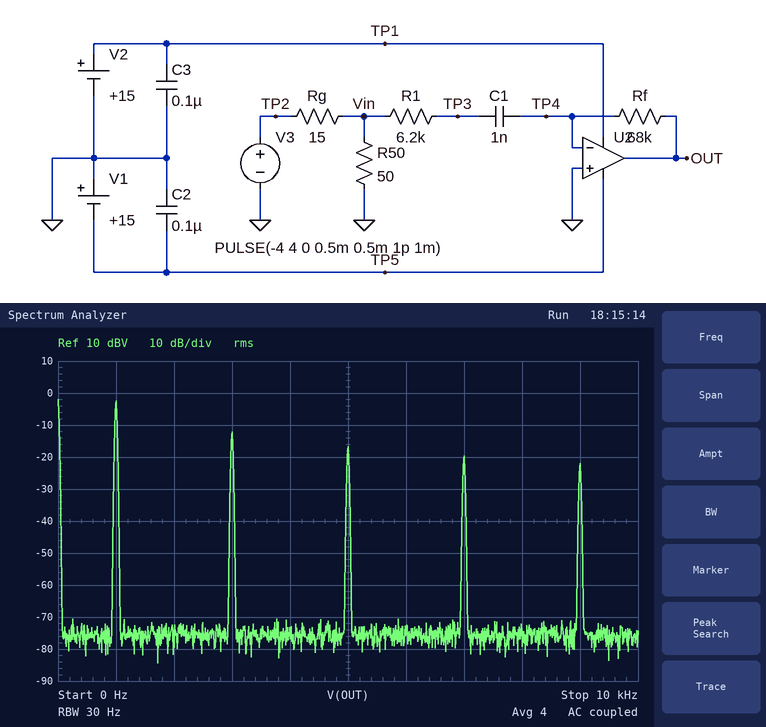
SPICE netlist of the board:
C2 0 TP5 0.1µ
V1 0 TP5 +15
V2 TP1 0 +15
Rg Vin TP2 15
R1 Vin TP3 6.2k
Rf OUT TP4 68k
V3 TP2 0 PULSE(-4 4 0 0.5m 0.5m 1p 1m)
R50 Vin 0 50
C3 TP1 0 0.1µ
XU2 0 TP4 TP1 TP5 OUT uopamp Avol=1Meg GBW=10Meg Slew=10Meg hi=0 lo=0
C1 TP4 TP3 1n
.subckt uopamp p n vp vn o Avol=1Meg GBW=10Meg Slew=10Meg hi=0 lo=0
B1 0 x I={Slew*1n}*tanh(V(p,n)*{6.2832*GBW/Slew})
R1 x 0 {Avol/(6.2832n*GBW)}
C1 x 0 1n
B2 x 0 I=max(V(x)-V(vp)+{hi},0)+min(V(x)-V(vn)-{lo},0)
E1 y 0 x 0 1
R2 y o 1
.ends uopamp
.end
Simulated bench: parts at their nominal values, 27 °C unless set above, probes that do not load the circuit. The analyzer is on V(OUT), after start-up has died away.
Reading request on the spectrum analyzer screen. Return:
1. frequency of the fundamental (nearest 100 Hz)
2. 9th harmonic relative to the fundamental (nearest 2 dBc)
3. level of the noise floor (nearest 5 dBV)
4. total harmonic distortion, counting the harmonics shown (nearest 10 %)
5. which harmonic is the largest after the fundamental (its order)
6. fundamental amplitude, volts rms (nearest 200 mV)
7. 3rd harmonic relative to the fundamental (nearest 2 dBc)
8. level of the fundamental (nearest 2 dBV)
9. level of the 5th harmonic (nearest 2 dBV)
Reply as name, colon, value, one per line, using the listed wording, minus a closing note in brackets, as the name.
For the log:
frequency of the fundamental: 1.0 kHz
9th harmonic relative to the fundamental: -20 dBc
level of the noise floor: -75 dBV
total harmonic distortion, counting the harmonics shown: 40 %
which harmonic is the largest after the fundamental: 3
fundamental amplitude, volts rms: 800 mV
3rd harmonic relative to the fundamental: -10 dBc
level of the fundamental: -2 dBV
level of the 5th harmonic: -16 dBV
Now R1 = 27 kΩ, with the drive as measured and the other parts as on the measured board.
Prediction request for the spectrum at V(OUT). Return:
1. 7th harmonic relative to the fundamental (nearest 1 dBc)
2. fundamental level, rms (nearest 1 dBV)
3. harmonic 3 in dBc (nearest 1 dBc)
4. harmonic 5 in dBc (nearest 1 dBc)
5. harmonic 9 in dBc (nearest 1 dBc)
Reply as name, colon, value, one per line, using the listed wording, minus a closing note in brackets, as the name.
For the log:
7th harmonic relative to the fundamental: -21 dBc
fundamental level, rms: -3 dBV
harmonic 3 in dBc: -10 dBc
harmonic 5 in dBc: -16 dBc
harmonic 9 in dBc: -24 dBc
